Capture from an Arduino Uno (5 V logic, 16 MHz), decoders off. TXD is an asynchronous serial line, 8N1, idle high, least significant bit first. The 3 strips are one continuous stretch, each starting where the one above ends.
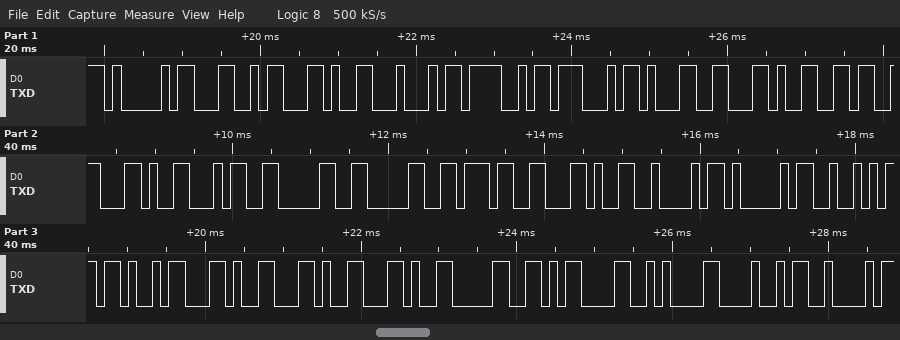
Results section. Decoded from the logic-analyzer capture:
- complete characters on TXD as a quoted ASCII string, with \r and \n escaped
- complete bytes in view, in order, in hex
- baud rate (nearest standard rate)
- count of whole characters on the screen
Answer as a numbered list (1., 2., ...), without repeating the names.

1. "AL,DOG1,6,4007,BARK,,,0\r\nHB"
2. 41 4C 2C 44 4F 47 31 2C 36 2C 34 30 30 37 2C 42 41 52 4B 2C 2C 2C 30 0D 0A 48 42
3. 9600 baud
4. 27
